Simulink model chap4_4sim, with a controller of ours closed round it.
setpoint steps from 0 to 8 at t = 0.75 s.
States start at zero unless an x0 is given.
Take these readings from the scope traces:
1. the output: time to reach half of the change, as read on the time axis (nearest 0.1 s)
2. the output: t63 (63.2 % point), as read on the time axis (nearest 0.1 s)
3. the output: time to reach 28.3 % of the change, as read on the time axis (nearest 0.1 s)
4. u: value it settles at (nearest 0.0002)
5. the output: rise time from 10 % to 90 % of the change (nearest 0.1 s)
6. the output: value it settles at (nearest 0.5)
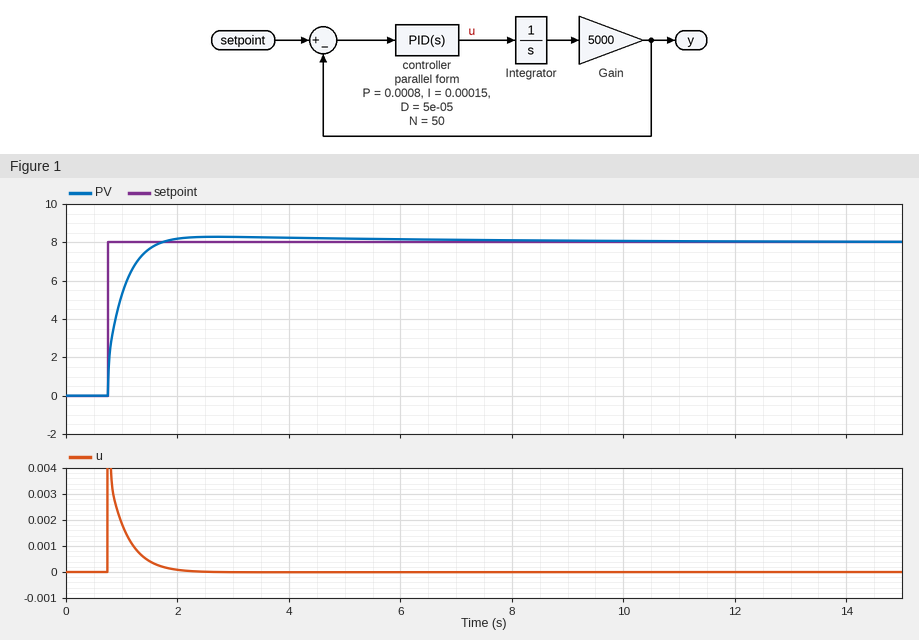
0.9 s
1.0 s
0.8 s
0.0000
0.6 s
8.0
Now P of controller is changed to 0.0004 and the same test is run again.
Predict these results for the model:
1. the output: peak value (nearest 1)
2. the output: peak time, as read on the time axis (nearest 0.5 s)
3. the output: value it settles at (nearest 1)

9
3.5 s
8
